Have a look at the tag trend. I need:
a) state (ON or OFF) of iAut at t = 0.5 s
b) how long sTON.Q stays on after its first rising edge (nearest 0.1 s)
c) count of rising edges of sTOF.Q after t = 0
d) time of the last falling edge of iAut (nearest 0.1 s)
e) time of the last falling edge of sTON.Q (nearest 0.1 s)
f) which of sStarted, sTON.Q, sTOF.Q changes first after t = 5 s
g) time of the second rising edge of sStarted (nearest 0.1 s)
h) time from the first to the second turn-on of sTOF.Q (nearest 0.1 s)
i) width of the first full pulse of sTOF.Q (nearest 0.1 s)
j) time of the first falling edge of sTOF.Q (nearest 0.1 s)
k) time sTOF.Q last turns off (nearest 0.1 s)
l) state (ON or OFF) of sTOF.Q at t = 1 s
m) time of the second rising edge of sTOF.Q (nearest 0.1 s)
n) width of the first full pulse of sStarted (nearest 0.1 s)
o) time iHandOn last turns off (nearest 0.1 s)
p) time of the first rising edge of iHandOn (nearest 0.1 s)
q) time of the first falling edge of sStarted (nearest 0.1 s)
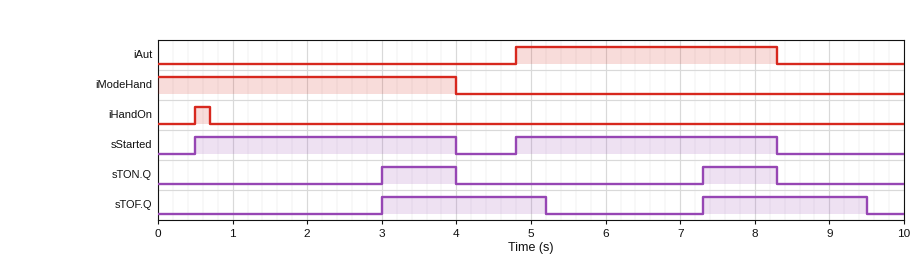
OFF
1.0 s
2
8.3 s
8.3 s
sTOF.Q
4.8 s
4.3 s
2.2 s
5.2 s
9.5 s
OFF
7.3 s
3.5 s
0.7 s
0.5 s
4.0 s
